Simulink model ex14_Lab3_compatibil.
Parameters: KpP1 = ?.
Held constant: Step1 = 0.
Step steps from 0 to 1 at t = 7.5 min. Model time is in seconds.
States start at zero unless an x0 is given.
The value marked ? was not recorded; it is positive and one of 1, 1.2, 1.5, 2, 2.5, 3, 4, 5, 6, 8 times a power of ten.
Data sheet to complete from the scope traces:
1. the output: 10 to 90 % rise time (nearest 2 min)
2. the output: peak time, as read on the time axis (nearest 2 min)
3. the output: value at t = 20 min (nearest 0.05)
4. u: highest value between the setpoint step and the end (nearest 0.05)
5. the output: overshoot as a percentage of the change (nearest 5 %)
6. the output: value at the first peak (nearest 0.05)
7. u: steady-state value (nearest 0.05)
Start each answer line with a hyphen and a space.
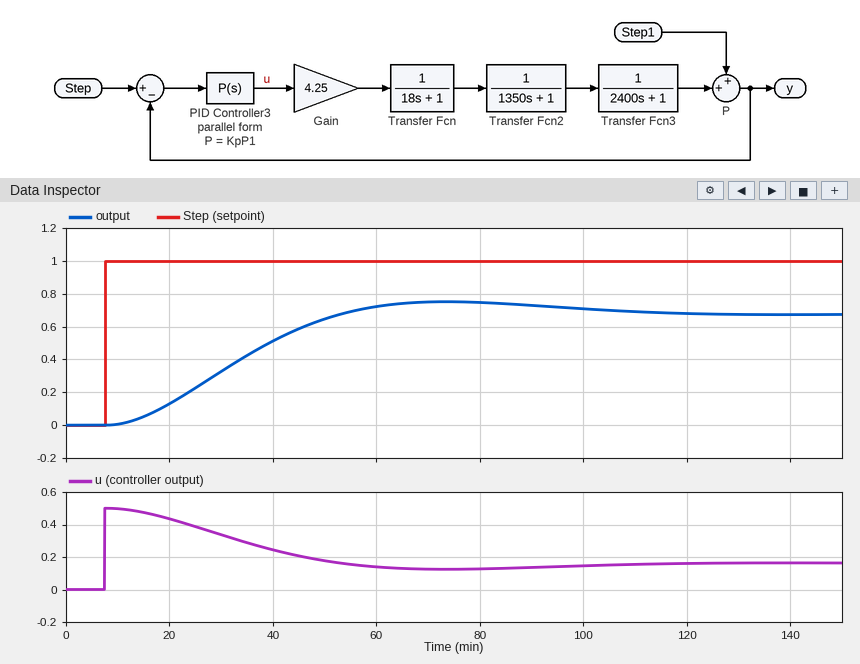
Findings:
- 30 min
- 74 min
- 0.15
- 0.50
- 10 %
- 0.75
- 0.15
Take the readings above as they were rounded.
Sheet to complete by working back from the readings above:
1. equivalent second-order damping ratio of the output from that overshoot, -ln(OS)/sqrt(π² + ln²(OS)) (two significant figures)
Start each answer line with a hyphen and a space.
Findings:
- 0.59
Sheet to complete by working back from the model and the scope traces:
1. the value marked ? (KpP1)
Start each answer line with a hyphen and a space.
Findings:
- 0.5
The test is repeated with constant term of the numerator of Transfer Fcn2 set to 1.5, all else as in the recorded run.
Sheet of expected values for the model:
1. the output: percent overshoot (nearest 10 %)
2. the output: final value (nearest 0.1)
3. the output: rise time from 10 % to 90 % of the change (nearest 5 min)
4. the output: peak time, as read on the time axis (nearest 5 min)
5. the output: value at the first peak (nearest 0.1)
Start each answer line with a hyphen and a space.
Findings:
- 20 %
- 0.8
- 25 min
- 60 min
- 0.9
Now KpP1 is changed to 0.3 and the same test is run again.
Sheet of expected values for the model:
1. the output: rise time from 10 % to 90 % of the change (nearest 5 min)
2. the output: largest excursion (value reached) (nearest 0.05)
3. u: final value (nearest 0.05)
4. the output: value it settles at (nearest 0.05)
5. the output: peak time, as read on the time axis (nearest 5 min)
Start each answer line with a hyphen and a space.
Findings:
- 40 min
- 0.60
- 0.15
- 0.55
- 95 min
